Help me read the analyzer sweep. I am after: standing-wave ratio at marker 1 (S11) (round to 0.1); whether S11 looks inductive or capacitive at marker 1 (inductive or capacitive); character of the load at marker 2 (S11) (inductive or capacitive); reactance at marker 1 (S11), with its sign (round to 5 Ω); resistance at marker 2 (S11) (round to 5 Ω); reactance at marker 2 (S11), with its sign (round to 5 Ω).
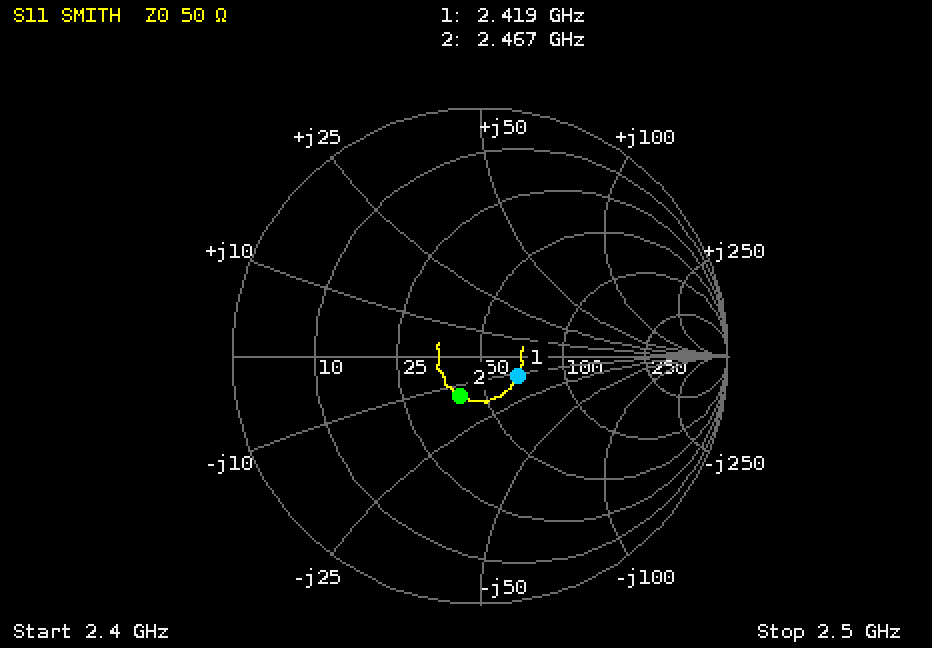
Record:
1.4
capacitive
capacitive
-10 Ω
40 Ω
-15 Ω
